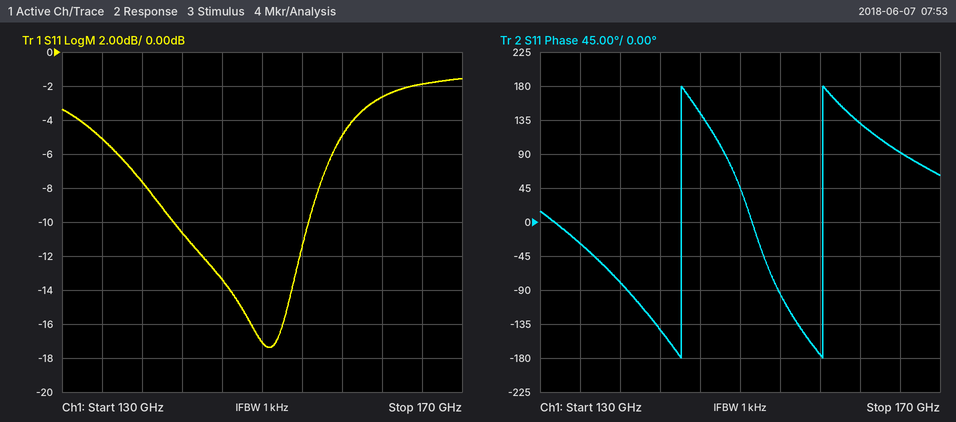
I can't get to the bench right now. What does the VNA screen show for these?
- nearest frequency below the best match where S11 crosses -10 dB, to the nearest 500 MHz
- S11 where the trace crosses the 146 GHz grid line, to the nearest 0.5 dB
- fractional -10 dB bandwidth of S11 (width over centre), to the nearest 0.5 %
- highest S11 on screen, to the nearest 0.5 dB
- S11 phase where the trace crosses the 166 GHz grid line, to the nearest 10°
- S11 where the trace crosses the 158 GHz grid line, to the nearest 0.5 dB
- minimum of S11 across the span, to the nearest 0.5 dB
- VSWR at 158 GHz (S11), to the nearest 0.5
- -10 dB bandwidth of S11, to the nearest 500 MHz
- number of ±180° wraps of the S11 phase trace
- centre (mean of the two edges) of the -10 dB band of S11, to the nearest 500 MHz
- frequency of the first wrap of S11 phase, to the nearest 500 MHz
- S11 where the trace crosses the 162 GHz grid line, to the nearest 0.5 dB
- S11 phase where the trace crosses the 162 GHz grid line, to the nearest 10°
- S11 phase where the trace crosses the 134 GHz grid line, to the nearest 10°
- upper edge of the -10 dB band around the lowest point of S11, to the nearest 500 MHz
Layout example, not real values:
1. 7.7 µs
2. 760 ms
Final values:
1. 141.0 GHz
2. -13.5 dB
3. 9.0 %
4. -1.5 dB
5. 90°
6. -5.0 dB
7. -17.5 dB
8. 3.5
9. 13.5 GHz
10. 2
11. 148.0 GHz
12. 144.0 GHz
13. -2.5 dB
14. 130°
15. -30°
16. 154.5 GHz
